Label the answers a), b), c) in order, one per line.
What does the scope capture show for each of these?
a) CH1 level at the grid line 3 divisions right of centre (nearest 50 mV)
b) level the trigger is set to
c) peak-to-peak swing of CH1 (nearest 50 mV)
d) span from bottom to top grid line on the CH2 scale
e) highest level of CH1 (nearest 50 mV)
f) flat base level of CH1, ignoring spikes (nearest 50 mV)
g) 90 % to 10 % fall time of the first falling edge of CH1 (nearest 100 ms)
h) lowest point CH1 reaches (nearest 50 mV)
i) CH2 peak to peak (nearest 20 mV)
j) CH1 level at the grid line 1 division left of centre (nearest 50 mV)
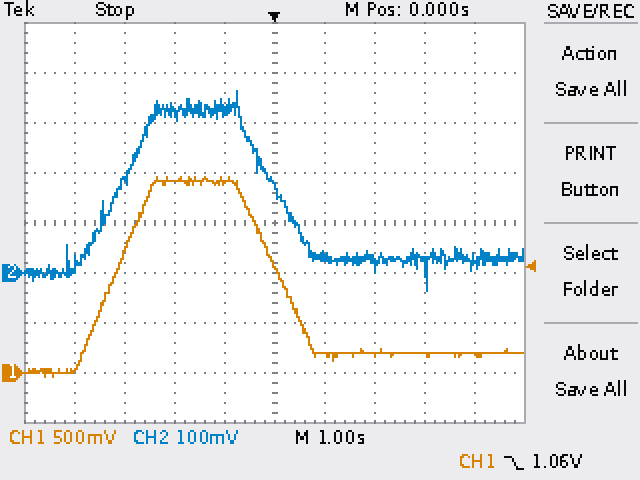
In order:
a) 200 mV
b) 1.06 V
c) 2.00 V
d) 800 mV
e) 1.95 V
f) 200 mV
g) 1.3 s
h) -50 mV
i) 400 mV
j) 1.90 V
